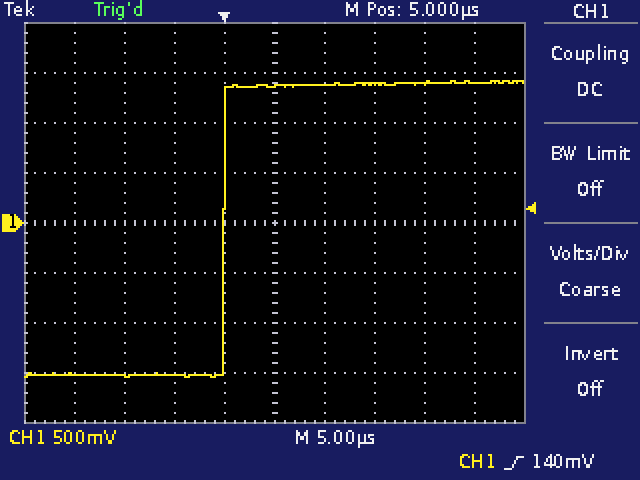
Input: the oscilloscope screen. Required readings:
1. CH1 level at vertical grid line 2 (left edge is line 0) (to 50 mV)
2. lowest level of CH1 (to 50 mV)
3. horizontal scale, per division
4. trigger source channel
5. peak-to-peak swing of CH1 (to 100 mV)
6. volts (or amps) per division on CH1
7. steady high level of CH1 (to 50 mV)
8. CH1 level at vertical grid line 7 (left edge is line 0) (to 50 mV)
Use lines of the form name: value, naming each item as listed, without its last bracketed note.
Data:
CH1 level at vertical grid line 2 (left edge is line 0): -1.55 V
lowest level of CH1: -1.55 V
horizontal scale, per division: 5 µs
trigger source channel: CH1
peak-to-peak swing of CH1: 3.00 V
volts (or amps) per division on CH1: 500 mV
steady high level of CH1: 1.40 V
CH1 level at vertical grid line 7 (left edge is line 0): 1.40 V
